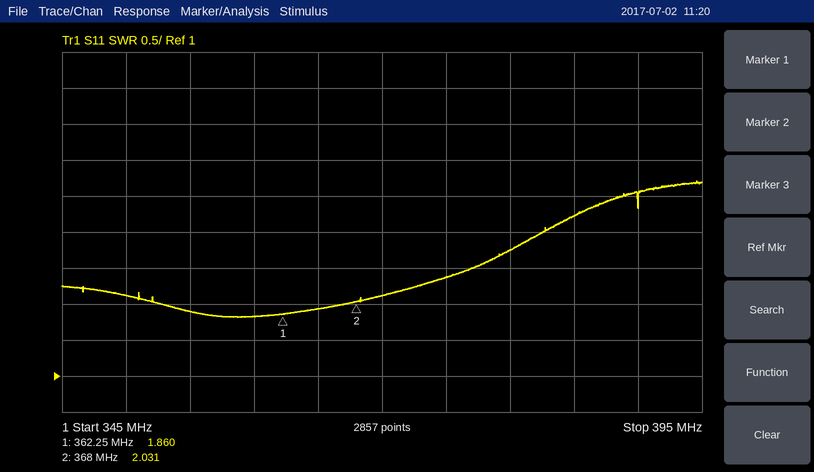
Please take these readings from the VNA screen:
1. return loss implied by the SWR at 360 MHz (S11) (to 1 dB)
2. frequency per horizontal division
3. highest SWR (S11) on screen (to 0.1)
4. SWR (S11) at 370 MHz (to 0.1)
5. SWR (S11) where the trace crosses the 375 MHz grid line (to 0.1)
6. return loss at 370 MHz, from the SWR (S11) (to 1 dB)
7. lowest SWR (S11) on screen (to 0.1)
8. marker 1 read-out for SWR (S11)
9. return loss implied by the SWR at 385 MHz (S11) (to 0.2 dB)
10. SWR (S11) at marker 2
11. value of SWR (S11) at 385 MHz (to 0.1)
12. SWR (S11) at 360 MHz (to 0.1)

11 dB
5 MHz
3.7
2.1
2.4
9 dB
1.8
1.860
5.6 dB
2.031
3.2
1.8
